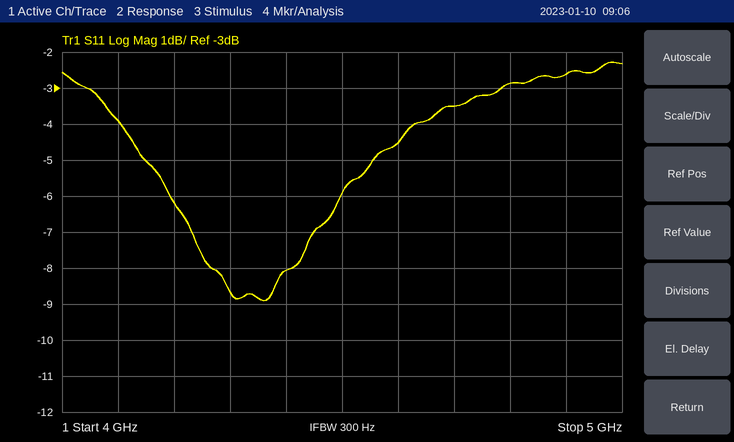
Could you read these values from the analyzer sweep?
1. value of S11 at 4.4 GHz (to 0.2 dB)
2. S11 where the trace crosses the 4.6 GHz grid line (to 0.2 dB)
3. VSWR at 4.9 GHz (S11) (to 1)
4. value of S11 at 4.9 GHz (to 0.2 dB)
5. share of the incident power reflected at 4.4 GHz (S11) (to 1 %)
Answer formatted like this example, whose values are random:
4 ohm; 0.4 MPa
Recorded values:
-8.0 dB; -4.6 dB; 7; -2.6 dB; 16 %
